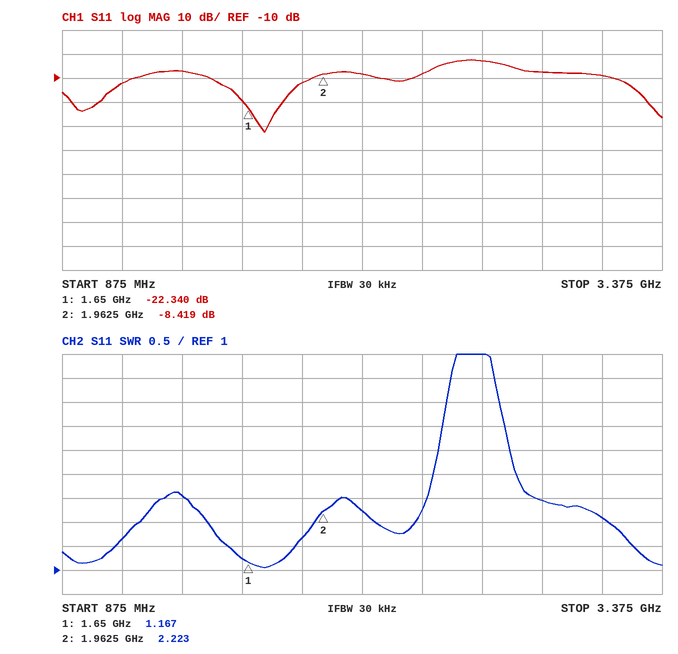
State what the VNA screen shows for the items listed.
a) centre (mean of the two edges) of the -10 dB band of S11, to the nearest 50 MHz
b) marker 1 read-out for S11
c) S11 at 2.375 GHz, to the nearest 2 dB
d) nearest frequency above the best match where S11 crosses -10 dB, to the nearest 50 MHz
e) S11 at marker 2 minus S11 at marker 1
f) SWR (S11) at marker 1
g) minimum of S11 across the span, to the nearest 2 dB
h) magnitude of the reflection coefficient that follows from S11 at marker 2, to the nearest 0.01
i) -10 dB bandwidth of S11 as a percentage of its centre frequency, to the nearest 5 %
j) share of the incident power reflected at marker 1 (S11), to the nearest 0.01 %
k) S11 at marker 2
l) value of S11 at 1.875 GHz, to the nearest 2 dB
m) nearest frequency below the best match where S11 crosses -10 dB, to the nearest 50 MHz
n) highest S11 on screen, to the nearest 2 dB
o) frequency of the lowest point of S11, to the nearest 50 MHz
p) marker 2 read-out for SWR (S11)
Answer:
1.70 GHz
-22.340 dB
-8 dB
1.90 GHz
13.921 dB
1.167
-32 dB
0.38
25 %
0.58 %
-8.419 dB
-12 dB
1.50 GHz
-2 dB
1.70 GHz
2.223
